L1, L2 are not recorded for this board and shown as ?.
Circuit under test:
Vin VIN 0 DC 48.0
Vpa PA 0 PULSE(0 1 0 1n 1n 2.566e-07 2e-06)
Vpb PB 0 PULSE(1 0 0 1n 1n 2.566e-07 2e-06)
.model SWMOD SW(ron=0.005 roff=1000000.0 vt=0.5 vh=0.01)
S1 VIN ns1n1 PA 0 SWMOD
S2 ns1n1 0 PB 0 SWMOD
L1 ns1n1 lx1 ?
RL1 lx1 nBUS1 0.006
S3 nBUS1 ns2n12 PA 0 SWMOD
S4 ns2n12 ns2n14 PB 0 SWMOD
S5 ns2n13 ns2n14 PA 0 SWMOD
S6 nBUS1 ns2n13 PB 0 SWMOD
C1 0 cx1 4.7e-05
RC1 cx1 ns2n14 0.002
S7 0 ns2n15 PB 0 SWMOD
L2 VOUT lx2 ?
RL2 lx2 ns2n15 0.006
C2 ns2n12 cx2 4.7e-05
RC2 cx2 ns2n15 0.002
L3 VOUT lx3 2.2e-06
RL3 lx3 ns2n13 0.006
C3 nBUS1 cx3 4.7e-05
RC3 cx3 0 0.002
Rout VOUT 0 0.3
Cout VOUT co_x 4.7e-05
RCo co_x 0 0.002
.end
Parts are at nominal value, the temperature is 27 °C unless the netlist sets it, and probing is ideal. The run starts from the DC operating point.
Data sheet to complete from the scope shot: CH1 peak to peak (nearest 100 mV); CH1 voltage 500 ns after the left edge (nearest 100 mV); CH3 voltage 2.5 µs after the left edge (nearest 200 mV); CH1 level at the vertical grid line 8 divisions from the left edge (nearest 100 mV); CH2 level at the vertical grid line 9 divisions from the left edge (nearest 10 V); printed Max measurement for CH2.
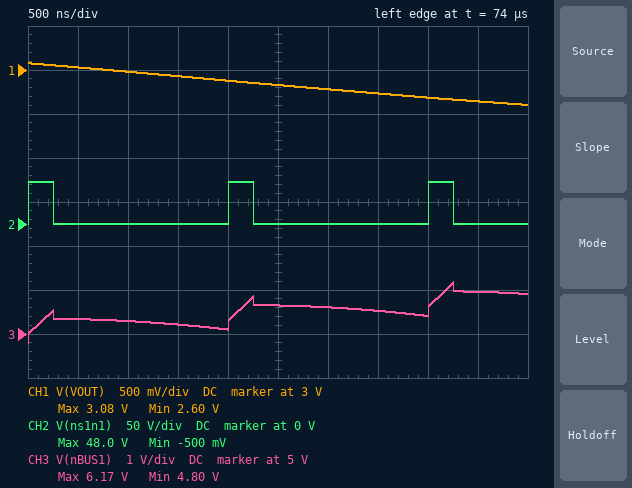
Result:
500 mV
3.0 V
5.6 V
2.7 V
0 V
48.0 V
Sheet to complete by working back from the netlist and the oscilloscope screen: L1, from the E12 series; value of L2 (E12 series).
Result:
1 µH
1.8 µH
